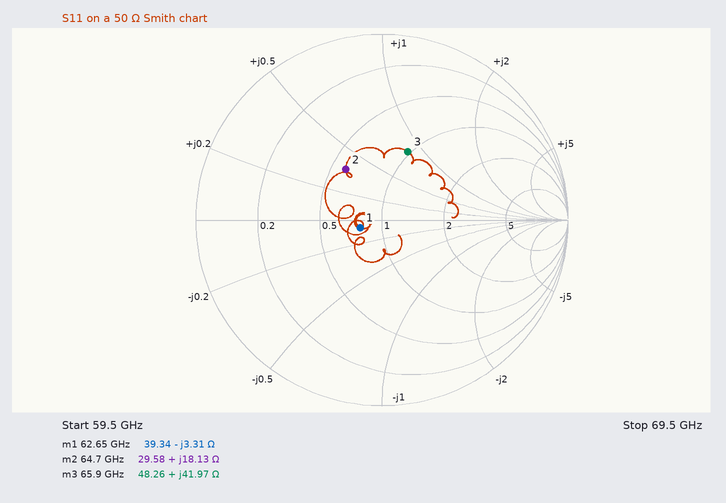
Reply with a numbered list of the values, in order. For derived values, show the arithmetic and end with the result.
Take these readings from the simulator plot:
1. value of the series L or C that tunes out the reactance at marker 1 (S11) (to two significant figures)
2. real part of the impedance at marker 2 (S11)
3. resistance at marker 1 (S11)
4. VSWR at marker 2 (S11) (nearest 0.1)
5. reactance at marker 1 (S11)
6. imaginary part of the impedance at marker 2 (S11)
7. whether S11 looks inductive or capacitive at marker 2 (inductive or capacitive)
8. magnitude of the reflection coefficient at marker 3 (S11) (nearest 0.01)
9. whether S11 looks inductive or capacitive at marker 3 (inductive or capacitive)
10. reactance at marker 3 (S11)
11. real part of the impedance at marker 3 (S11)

1. L = 3.31 Ω/(2π × 62.65 GHz) ≈ 8.4 pH
2. 29.58 Ω
3. 39.34 Ω
4. 2.0
5. -3.31 Ω
6. +18.13 Ω
7. inductive
8. 0.39
9. inductive
10. +41.97 Ω
11. 48.26 Ω
